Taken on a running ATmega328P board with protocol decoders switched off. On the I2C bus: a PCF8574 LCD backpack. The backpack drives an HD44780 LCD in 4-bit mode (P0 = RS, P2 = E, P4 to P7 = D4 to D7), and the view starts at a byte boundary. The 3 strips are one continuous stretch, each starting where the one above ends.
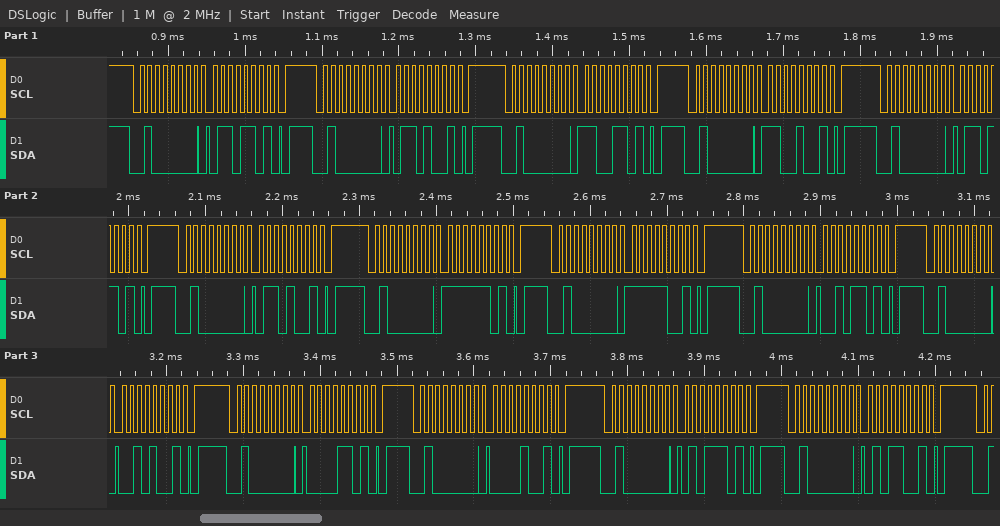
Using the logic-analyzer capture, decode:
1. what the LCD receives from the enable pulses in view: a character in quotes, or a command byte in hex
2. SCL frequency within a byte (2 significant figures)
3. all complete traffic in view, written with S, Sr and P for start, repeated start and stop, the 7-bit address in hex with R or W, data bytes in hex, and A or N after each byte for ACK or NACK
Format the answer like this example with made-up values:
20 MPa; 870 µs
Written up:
'l' 'o' ' '; 100 kHz; S 20W A 6D A P S 20W A 69 A P S 20W A CD A P S 20W A C9 A P S 20W A 6D A P S 20W A 69 A P S 20W A FD A P S 20W A F9 A P S 20W A 2D A P S 20W A 29 A P S 20W A 0D A P S 20W A 09 A P S 20W A 5D A P S 20W A 59 A P
